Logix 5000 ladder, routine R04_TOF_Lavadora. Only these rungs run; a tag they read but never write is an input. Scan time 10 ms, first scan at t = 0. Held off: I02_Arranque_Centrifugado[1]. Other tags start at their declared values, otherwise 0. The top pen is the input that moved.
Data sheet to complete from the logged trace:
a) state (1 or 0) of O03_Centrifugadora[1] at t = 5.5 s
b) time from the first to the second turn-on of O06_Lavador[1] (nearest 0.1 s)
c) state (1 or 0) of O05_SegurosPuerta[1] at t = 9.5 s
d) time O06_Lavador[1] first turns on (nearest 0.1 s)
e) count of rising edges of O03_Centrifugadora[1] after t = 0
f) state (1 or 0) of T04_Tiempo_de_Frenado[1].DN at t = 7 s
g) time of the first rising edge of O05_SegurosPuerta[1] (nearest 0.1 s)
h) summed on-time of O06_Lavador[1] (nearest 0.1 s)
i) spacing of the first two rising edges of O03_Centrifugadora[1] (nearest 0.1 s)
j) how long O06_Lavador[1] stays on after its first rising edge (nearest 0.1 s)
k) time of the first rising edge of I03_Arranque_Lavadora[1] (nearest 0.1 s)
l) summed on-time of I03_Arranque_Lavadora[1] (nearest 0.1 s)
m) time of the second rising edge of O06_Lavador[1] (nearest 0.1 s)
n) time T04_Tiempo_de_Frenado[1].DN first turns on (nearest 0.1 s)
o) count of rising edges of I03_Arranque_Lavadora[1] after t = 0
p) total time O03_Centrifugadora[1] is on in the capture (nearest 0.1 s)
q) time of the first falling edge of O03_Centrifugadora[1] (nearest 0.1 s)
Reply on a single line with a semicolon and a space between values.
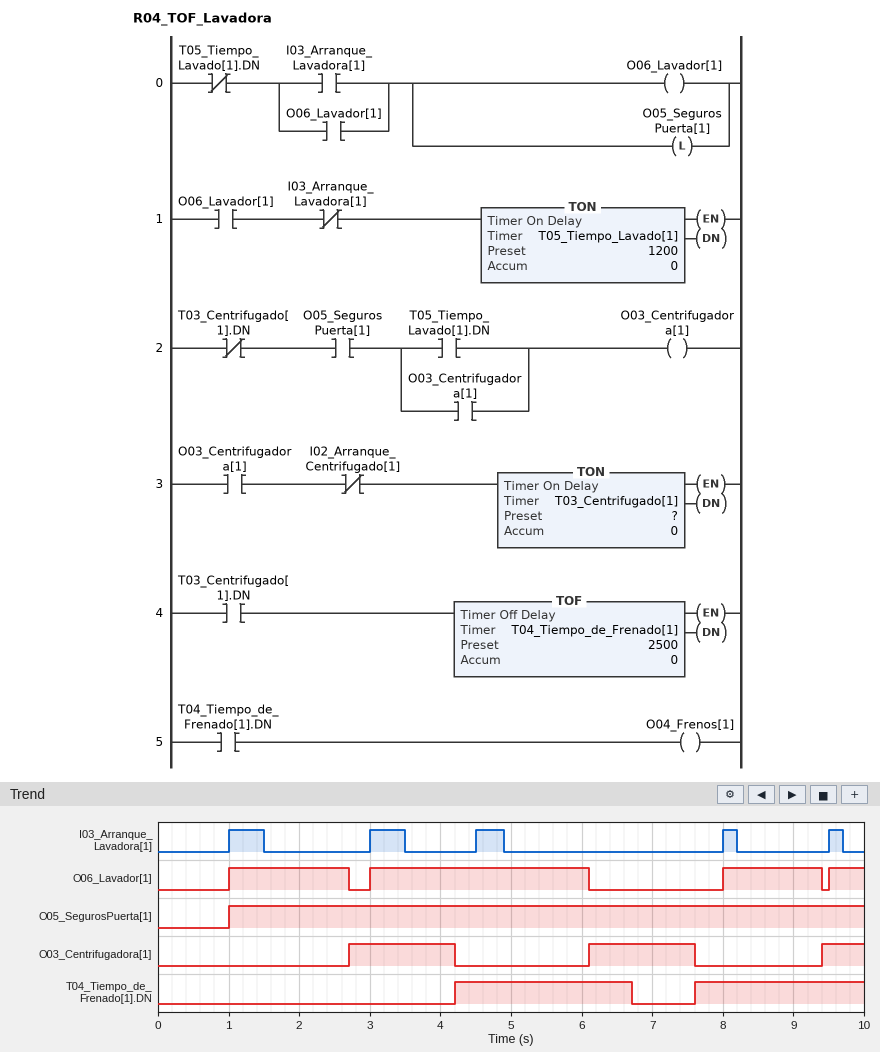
0; 2.0 s; 1; 1.0 s; 3; 0; 1.0 s; 6.7 s; 3.4 s; 1.7 s; 1.0 s; 1.8 s; 3.0 s; 4.2 s; 5; 3.6 s; 4.2 s
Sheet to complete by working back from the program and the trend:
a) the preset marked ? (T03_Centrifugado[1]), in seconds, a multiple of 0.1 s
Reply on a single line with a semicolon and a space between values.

1.5 s
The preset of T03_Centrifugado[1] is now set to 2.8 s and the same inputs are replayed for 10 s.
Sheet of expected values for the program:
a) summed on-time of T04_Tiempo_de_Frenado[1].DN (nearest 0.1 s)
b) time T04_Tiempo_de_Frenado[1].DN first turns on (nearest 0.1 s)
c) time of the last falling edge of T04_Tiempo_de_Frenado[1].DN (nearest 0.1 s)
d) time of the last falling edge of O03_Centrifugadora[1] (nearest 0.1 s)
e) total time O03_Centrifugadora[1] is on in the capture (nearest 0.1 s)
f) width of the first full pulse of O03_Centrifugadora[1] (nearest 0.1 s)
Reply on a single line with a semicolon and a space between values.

3.6 s; 5.5 s; 8.0 s; 8.9 s; 6.2 s; 2.8 s
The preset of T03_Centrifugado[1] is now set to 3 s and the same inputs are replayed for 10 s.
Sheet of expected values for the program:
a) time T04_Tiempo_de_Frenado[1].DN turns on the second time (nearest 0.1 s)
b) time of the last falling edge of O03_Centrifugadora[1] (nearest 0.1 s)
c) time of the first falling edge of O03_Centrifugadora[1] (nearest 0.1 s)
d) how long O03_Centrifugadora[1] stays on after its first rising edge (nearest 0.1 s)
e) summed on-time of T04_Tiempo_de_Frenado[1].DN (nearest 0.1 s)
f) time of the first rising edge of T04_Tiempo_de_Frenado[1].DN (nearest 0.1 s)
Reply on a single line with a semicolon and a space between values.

9.1 s; 9.1 s; 5.7 s; 3.0 s; 3.4 s; 5.7 s
